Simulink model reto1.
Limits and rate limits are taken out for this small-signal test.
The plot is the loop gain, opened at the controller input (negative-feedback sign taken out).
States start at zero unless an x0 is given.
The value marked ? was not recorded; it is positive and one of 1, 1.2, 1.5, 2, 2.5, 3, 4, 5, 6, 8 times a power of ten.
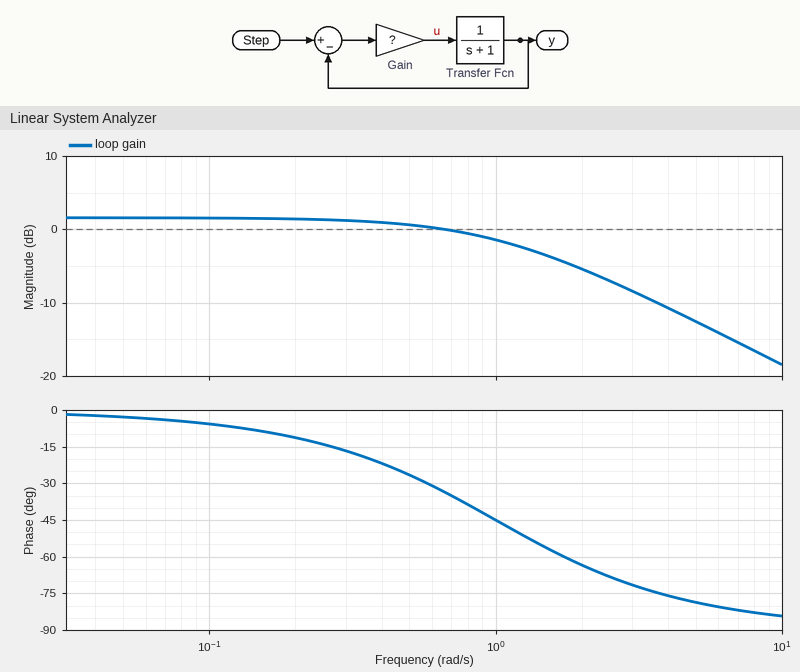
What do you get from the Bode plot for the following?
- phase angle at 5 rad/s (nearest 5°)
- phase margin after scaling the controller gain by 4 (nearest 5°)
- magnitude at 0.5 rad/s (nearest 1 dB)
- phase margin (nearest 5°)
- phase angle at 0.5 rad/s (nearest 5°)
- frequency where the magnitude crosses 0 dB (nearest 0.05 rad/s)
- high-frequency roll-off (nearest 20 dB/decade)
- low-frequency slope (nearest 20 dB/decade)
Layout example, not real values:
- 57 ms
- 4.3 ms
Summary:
- -80°
- 100°
- 1 dB
- 145°
- -25°
- 0.65 rad/s
- -20 dB/decade
- 0 dB/decade
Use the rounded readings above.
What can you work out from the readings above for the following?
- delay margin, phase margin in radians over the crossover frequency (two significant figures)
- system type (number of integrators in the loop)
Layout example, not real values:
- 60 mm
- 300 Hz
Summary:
- 3.9 s
- 0
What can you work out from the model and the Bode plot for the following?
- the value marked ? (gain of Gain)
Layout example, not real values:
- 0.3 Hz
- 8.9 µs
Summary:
- 1.2
